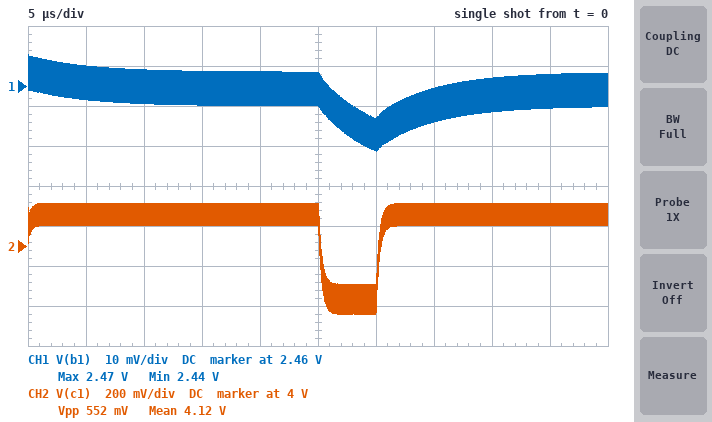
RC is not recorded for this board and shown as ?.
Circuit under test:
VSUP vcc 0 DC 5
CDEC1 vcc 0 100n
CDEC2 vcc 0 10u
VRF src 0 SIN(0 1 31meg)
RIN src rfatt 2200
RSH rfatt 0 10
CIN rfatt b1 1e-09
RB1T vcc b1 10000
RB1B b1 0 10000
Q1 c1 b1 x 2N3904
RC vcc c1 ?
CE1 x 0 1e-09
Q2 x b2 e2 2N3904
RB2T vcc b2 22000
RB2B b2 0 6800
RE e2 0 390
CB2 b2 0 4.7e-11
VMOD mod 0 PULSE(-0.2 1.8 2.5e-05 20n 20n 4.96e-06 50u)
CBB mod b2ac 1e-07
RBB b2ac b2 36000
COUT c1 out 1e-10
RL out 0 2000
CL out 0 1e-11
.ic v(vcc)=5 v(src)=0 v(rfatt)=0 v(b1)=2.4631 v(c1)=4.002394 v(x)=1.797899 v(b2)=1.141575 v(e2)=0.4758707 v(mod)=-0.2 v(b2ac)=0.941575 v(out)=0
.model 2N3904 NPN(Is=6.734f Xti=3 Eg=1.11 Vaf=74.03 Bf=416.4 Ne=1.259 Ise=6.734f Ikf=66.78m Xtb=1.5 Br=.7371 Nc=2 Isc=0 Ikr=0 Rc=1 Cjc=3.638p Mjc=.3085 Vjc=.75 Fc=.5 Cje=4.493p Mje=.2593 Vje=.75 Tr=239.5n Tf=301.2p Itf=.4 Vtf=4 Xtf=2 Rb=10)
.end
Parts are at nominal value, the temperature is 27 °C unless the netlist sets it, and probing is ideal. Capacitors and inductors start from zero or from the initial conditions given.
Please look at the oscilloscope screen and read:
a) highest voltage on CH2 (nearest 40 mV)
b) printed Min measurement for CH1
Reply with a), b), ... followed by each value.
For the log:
a) 4.20 V
b) 2.44 V
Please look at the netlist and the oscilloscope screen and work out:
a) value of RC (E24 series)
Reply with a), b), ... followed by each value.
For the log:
a) 750 Ω
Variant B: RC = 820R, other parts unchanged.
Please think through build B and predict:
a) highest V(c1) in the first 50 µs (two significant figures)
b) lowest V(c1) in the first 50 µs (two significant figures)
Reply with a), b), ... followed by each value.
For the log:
a) 4.1 V
b) 3.5 V
